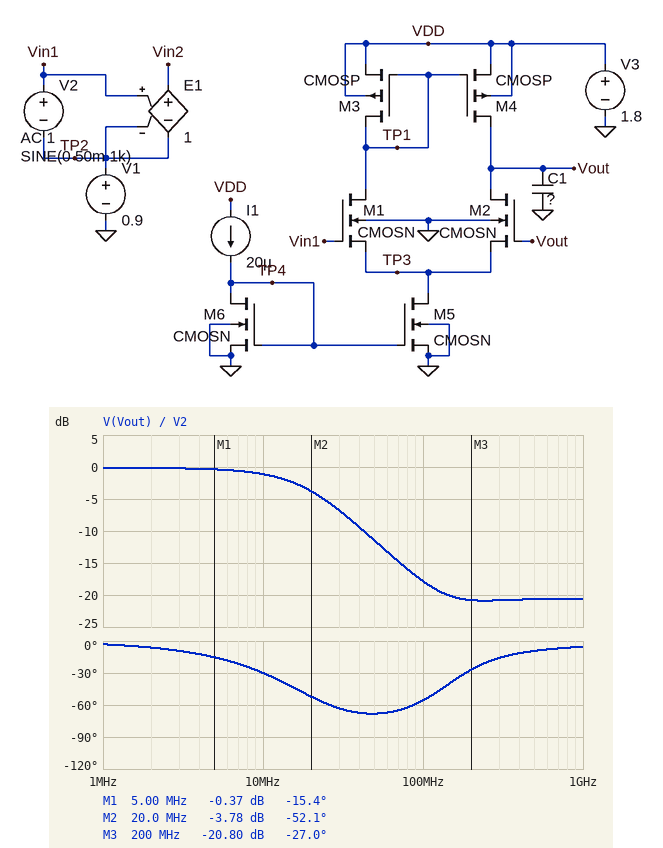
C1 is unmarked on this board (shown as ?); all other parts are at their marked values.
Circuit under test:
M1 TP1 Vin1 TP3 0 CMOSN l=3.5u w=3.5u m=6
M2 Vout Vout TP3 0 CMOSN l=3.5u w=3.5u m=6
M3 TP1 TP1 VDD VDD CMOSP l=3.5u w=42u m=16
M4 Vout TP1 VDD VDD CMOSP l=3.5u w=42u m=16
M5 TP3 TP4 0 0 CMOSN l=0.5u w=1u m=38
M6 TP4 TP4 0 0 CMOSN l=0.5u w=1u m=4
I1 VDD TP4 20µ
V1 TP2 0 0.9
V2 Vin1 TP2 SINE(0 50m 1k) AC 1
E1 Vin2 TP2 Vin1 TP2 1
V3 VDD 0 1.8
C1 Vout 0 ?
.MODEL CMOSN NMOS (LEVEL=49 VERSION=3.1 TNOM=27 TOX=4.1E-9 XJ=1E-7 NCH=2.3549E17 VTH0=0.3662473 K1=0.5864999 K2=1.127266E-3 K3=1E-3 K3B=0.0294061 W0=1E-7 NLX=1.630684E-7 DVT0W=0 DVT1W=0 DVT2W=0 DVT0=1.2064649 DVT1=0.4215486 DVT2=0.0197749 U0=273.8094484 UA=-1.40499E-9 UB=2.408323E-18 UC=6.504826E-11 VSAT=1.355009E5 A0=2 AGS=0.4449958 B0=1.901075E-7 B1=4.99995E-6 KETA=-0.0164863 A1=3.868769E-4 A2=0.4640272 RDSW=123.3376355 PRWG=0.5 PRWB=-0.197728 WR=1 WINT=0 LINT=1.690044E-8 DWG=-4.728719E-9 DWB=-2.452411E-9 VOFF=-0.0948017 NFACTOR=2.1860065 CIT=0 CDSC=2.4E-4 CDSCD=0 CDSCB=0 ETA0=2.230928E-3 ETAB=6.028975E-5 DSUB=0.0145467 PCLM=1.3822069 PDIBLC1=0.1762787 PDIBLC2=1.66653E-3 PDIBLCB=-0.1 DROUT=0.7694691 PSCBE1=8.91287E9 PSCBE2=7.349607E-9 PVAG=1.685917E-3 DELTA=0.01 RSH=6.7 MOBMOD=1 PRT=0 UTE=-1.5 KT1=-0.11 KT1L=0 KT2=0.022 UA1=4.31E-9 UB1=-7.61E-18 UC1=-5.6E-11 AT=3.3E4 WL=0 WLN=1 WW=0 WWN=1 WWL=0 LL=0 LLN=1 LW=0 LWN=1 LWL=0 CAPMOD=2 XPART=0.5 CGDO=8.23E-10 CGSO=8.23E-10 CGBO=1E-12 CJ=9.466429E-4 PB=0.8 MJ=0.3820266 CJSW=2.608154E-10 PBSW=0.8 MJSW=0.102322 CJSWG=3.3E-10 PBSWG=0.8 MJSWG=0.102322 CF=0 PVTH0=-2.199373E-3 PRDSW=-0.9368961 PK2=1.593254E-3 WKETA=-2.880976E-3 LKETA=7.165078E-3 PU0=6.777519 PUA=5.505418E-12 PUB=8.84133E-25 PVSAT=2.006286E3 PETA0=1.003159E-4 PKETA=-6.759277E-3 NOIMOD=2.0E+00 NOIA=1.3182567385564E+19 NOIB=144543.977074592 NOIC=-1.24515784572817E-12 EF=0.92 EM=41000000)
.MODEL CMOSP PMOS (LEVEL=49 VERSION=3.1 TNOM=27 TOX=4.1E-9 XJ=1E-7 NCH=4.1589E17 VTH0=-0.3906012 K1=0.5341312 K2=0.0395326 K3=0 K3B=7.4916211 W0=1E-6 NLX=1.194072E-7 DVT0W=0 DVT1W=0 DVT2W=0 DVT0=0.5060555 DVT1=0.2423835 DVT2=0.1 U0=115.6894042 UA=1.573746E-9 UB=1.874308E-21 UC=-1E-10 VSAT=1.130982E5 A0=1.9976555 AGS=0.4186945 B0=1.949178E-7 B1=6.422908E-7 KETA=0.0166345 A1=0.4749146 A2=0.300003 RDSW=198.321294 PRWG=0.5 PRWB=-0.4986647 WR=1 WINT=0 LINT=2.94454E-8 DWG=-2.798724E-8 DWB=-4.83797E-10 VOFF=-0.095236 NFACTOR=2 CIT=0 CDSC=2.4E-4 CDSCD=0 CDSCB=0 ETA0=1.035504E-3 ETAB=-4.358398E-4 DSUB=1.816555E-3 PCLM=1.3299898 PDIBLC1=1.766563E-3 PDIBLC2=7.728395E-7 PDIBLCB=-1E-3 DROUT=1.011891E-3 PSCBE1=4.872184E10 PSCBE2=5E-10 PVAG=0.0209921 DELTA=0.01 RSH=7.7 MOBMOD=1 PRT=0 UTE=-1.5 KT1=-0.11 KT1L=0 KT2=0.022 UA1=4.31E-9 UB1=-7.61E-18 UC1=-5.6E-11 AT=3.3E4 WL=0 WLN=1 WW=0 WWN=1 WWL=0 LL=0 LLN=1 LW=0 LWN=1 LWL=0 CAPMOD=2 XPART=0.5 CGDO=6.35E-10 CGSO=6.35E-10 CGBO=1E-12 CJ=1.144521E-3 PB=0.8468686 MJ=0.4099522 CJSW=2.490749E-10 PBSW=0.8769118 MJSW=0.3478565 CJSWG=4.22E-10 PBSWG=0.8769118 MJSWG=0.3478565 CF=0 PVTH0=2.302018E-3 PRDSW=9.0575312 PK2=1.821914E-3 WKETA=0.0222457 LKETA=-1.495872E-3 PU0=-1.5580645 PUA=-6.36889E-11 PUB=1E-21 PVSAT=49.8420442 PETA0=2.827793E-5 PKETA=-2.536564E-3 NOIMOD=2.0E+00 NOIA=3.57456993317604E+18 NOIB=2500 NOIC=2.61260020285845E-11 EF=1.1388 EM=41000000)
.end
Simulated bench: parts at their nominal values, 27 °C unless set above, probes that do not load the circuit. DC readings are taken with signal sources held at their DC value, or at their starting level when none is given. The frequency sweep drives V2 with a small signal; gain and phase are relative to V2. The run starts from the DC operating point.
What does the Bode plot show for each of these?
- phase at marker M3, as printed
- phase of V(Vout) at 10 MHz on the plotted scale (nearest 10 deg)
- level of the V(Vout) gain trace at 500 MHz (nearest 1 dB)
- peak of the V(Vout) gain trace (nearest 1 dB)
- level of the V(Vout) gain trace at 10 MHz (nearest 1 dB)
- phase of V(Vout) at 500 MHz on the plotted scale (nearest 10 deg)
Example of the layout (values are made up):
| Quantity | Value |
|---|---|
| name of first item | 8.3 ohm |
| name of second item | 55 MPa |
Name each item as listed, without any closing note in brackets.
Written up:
| Quantity | Value |
|---|---|
| phase at marker M3, as printed | -27.0 deg |
| phase of V(Vout) at 10 MHz on the plotted scale | -30 deg |
| level of the V(Vout) gain trace at 500 MHz | -21 dB |
| peak of the V(Vout) gain trace | 0 dB |
| level of the V(Vout) gain trace at 10 MHz | -1 dB |
| phase of V(Vout) at 500 MHz on the plotted scale | -10 deg |
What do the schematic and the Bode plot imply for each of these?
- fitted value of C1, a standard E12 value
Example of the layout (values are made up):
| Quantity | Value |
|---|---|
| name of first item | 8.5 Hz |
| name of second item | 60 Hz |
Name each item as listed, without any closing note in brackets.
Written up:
| Quantity | Value |
|---|---|
| fitted value of C1, a standard E12 value | 470 fF |
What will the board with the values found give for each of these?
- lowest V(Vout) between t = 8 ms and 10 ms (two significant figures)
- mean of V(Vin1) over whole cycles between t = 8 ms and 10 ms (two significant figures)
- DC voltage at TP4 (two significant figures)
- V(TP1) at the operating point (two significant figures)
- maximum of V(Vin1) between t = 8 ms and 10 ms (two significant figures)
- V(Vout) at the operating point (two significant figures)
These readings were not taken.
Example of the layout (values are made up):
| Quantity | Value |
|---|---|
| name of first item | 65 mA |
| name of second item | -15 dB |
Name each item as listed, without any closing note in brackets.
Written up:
| Quantity | Value |
|---|---|
| lowest V(Vout) between t = 8 ms and 10 ms | 860 mV |
| mean of V(Vin1) over whole cycles between t = 8 ms and 10 ms | 900 mV |
| DC voltage at TP4 | 570 mV |
| V(TP1) at the operating point | 1.3 V |
| maximum of V(Vin1) between t = 8 ms and 10 ms | 950 mV |
| V(Vout) at the operating point | 910 mV |
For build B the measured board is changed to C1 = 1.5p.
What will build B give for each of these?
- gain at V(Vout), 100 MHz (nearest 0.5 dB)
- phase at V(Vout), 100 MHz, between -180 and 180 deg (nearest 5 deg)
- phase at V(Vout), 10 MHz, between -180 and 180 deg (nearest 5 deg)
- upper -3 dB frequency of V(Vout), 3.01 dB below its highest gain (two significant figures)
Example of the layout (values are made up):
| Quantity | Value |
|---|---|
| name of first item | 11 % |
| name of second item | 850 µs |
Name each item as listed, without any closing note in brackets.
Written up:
| Quantity | Value |
|---|---|
| gain at V(Vout), 100 MHz | -22.5 dB |
| phase at V(Vout), 100 MHz, between -180 and 180 deg | -65 deg |
| phase at V(Vout), 10 MHz, between -180 and 180 deg | -40 deg |
| upper -3 dB frequency of V(Vout), 3.01 dB below its highest gain | 15 MHz |
